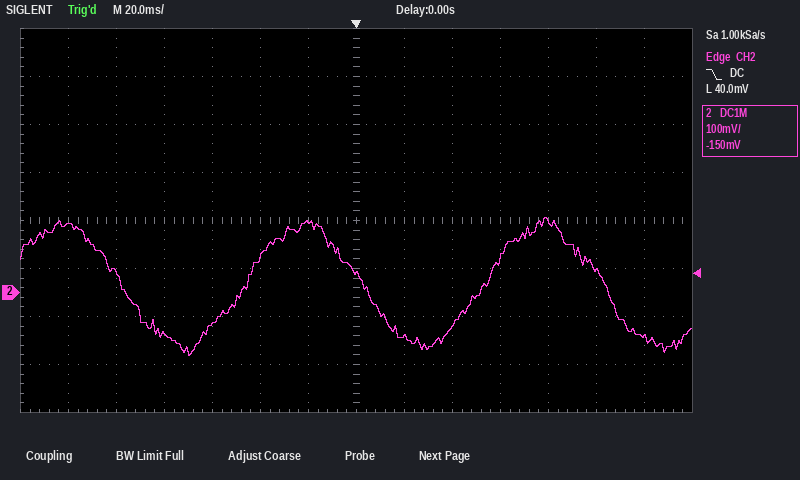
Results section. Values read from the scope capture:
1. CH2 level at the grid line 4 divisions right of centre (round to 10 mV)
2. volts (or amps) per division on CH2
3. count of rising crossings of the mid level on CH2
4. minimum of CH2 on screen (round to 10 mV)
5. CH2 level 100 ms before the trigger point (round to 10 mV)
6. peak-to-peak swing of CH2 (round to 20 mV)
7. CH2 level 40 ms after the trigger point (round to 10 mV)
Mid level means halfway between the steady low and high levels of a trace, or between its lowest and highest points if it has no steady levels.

150 mV
100 mV
2
-130 mV
40 mV
280 mV
-70 mV
